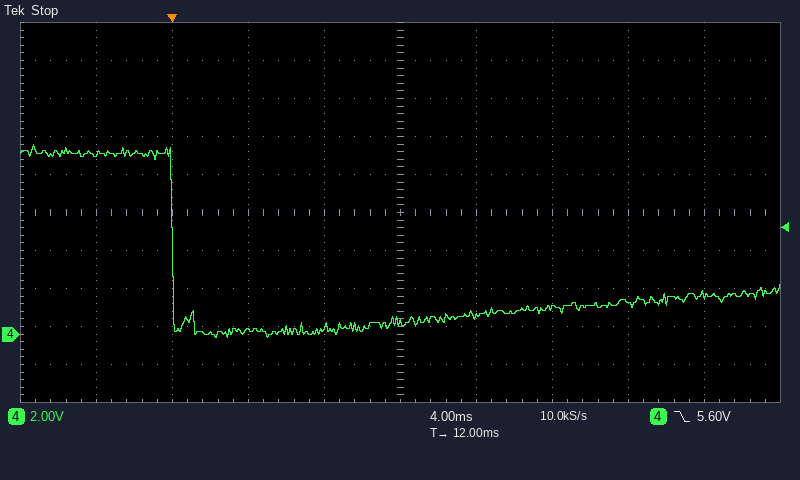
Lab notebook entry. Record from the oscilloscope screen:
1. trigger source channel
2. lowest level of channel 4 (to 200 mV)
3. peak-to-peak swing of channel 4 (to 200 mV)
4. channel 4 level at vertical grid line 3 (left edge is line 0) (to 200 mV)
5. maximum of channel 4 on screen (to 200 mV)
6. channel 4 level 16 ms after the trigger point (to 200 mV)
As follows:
channel 4
-200 mV
10.2 V
200 mV
10.0 V
1.0 V
